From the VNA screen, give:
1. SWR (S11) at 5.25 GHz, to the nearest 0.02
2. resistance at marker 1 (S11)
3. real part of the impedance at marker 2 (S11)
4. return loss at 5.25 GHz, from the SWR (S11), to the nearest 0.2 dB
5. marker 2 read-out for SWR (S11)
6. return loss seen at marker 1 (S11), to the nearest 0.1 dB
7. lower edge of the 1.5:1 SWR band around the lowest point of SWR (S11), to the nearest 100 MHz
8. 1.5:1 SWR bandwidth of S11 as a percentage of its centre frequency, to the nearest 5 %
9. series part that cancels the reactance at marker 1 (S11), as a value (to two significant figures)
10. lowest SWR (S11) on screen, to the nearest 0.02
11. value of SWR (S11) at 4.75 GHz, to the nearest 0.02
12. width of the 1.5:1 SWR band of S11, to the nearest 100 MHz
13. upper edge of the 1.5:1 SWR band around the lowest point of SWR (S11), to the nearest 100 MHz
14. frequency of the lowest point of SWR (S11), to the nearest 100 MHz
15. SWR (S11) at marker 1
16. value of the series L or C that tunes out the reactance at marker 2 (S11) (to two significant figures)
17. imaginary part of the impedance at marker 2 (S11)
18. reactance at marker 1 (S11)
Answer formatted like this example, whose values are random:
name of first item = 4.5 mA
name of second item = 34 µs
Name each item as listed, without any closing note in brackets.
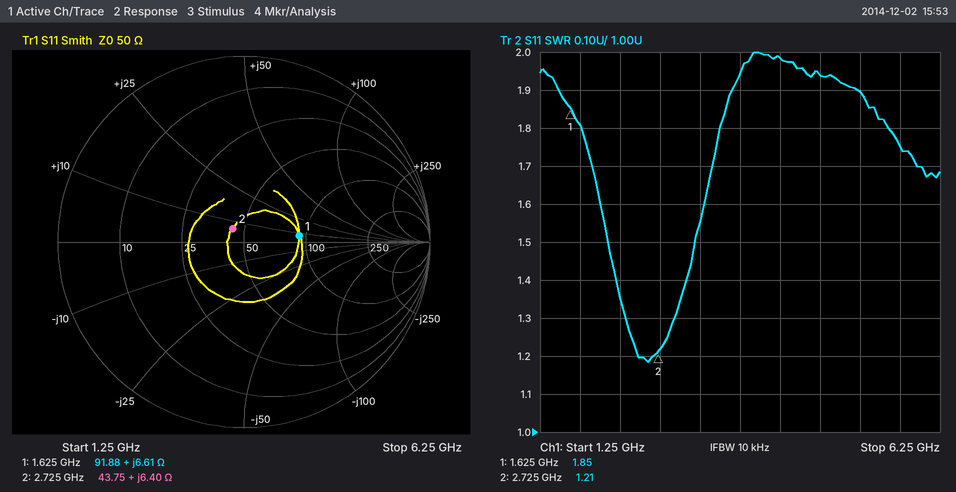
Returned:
SWR (S11) at 5.25 GHz, to the nearest 0.02 = 1.90
resistance at marker 1 = 91.88 Ω
real part of the impedance at marker 2 = 43.75 Ω
return loss at 5.25 GHz, from the SWR (S11), to the nearest 0.2 dB = 10.2 dB
marker 2 read-out for SWR = 1.21
return loss seen at marker 1 (S11), to the nearest 0.1 dB = 10.5 dB
lower edge of the 1.5:1 SWR band around the lowest point of SWR (S11), to the nearest 100 MHz = 2.1 GHz
1.5:1 SWR bandwidth of S11 as a percentage of its centre frequency, to the nearest 5 % = 40 %
series part that cancels the reactance at marker 1 (S11), as a value = 15 pF
lowest SWR (S11) on screen, to the nearest 0.02 = 1.18
value of SWR (S11) at 4.75 GHz, to the nearest 0.02 = 1.94
width of the 1.5:1 SWR band of S11, to the nearest 100 MHz = 1.1 GHz
upper edge of the 1.5:1 SWR band around the lowest point of SWR (S11), to the nearest 100 MHz = 3.2 GHz
frequency of the lowest point of SWR (S11), to the nearest 100 MHz = 2.6 GHz
SWR (S11) at marker 1 = 1.85
value of the series L or C that tunes out the reactance at marker 2 (S11) = 9.1 pF
imaginary part of the impedance at marker 2 = +6.40 Ω
reactance at marker 1 = +6.61 Ω
